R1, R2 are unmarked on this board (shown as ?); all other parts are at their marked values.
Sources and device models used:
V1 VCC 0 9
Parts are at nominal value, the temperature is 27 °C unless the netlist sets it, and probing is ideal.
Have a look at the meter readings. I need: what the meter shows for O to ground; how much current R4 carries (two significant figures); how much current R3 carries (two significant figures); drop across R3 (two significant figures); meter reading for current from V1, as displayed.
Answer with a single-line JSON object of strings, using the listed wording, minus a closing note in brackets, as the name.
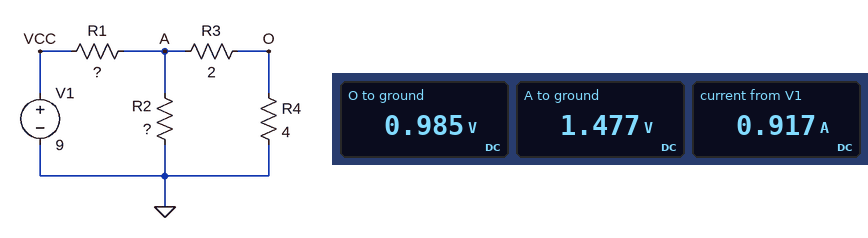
{"what the meter shows for O to ground": "0.985 V", "how much current R4 carries": "250 mA", "how much current R3 carries": "250 mA", "drop across R3": "490 mV", "meter reading for current from V1, as displayed": "0.917 A"}
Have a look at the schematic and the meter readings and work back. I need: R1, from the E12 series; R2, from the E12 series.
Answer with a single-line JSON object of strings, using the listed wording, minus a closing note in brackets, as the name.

{"R1, from the E12 series": "8.2 Ω", "R2, from the E12 series": "2.2 Ω"}
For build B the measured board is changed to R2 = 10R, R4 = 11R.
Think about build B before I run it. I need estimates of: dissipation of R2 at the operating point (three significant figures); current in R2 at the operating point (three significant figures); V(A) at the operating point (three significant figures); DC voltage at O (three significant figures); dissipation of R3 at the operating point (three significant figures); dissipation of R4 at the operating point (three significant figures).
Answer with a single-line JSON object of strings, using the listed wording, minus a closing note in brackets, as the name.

{"dissipation of R2 at the operating point": "1.35 W", "current in R2 at the operating point": "367 mA", "V(A) at the operating point": "3.67 V", "DC voltage at O": "3.11 V", "dissipation of R3 at the operating point": "160 mW", "dissipation of R4 at the operating point": "878 mW"}
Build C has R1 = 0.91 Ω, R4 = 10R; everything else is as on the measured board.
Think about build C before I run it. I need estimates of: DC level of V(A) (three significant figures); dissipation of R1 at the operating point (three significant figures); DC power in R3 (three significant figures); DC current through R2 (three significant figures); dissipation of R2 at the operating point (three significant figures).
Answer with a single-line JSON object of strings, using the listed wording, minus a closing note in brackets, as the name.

{"DC level of V(A)": "6.04 V", "dissipation of R1 at the operating point": "9.61 W", "DC power in R3": "507 mW", "DC current through R2": "2.75 A", "dissipation of R2 at the operating point": "16.6 W"}
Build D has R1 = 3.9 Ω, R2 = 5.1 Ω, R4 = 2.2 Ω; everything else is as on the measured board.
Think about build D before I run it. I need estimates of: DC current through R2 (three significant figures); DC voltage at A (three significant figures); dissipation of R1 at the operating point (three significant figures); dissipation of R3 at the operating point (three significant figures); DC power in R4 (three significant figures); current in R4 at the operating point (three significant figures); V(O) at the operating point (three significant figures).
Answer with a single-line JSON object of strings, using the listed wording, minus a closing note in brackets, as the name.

{"DC current through R2": "655 mA", "DC voltage at A": "3.34 V", "dissipation of R1 at the operating point": "8.21 W", "dissipation of R3 at the operating point": "1.27 W", "DC power in R4": "1.39 W", "current in R4 at the operating point": "796 mA", "V(O) at the operating point": "1.75 V"}
